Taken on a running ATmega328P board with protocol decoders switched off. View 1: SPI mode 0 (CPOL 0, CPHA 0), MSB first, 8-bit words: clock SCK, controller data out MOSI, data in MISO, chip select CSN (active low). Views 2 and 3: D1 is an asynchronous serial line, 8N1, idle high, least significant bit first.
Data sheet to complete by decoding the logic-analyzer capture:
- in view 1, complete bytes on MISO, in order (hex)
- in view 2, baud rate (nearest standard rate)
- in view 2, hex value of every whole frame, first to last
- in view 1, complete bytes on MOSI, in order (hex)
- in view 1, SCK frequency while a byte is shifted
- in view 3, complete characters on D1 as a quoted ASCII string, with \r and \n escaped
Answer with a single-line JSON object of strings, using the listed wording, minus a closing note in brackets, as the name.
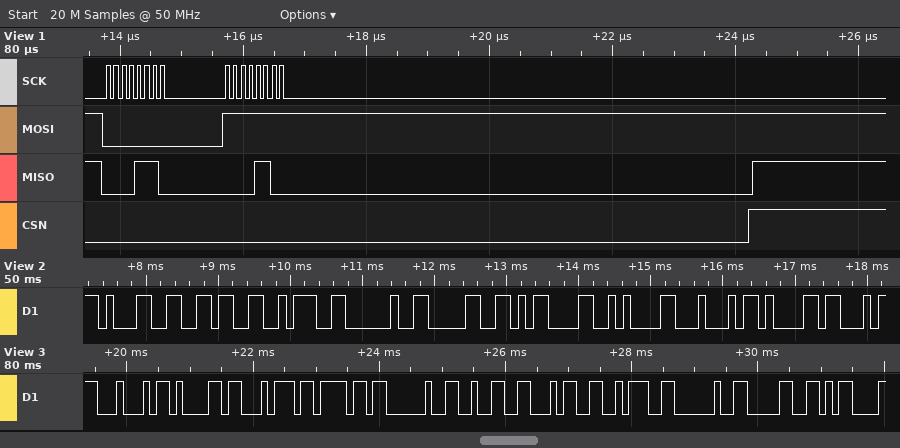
{"in view 1, complete bytes on MISO, in order": "0E 0C", "in view 2, baud rate": "9600 baud", "in view 2, hex value of every whole frame, first to last": "31 36 3A 20 30 0D 0A 44 61", "in view 1, complete bytes on MOSI, in order": "00 FF", "in view 1, SCK frequency while a byte is shifted": "8 MHz", "in view 3, complete characters on D1 as a quoted ASCII string, with \\r and \\n escaped": "\"Dato 24: 0\\r\""}
